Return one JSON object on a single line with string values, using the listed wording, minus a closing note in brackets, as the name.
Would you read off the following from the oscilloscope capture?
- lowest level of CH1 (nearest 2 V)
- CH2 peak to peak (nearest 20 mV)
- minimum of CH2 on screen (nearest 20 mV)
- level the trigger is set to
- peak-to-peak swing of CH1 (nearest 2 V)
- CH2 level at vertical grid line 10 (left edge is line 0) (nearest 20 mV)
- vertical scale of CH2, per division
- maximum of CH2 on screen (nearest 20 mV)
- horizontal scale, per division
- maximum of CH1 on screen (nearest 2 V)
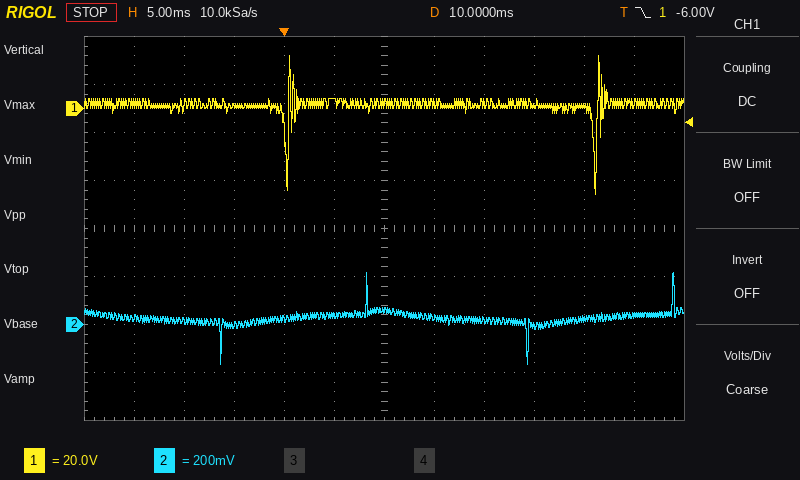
{"lowest level of CH1": "-36 V", "CH2 peak to peak": "380 mV", "minimum of CH2 on screen": "-160 mV", "level the trigger is set to": "-6.00 V", "peak-to-peak swing of CH1": "58 V", "CH2 level at vertical grid line 10 (left edge is line 0)": "20 mV", "vertical scale of CH2, per division": "200 mV", "maximum of CH2 on screen": "220 mV", "horizontal scale, per division": "5 ms", "maximum of CH1 on screen": "22 V"}
